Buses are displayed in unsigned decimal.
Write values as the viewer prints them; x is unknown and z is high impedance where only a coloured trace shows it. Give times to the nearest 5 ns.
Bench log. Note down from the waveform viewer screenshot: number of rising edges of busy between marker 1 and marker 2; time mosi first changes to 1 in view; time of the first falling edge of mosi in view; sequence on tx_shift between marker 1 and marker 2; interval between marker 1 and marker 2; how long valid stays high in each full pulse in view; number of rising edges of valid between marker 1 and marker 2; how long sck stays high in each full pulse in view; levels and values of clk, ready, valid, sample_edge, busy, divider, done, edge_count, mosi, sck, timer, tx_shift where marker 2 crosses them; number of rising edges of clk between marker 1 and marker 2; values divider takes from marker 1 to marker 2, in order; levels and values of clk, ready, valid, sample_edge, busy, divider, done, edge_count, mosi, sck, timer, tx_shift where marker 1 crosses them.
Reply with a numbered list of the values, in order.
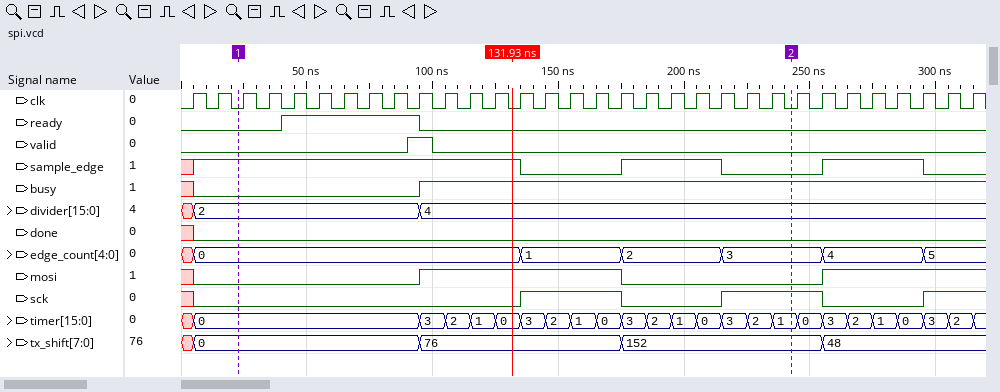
1. 1
2. 95 ns
3. 175 ns
4. 0, 76, 152
5. 220 ns
6. 10 ns
7. 1
8. 40 ns, 40 ns
9. clk=0, ready=0, valid=0, sample_edge=0, busy=1, divider=4, done=0, edge_count=3, mosi=0, sck=1, timer=1, tx_shift=152
10. 22
11. 2, 4
12. clk=0, ready=0, valid=0, sample_edge=1, busy=0, divider=2, done=0, edge_count=0, mosi=0, sck=0, timer=0, tx_shift=0
